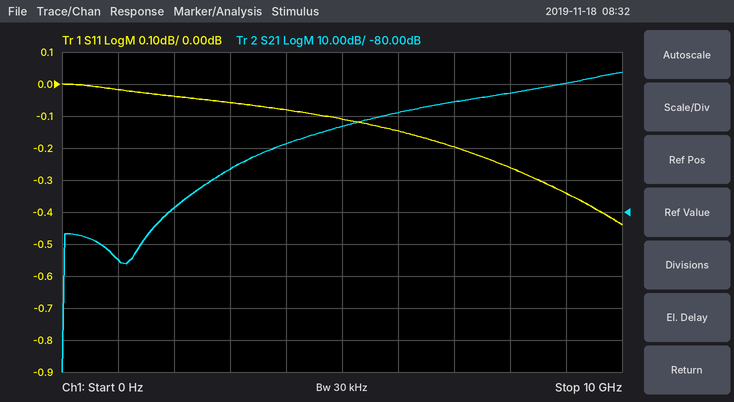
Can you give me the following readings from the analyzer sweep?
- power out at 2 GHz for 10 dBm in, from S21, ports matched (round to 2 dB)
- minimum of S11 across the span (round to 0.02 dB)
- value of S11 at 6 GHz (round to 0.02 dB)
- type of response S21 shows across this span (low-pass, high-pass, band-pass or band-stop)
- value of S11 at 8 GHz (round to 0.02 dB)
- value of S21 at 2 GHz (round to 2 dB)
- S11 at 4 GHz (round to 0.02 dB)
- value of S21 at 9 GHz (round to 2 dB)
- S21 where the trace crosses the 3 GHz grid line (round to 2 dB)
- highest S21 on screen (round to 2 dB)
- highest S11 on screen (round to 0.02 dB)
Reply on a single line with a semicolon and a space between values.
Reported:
-68 dBm; -0.44 dB; -0.14 dB; high-pass; -0.26 dB; -78 dB; -0.08 dB; -40 dB; -66 dB; -36 dB; 0.00 dB
